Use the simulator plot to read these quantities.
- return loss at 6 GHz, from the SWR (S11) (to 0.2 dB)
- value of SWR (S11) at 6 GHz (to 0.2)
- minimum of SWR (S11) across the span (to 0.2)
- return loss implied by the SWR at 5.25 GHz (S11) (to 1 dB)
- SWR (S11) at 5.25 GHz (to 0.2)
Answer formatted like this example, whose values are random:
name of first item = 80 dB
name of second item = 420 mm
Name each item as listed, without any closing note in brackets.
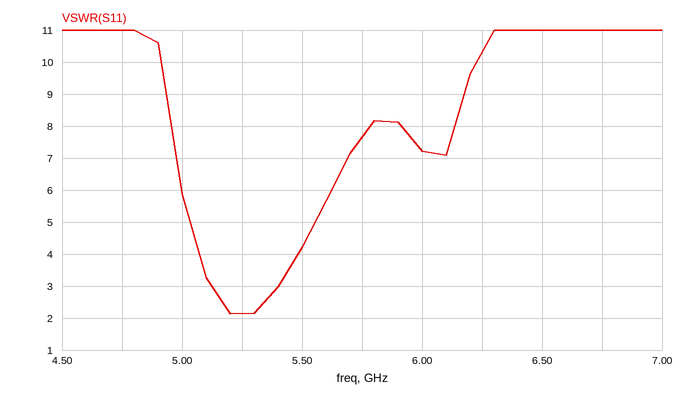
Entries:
return loss at 6 GHz, from the SWR (S11) = 2.4 dB
value of SWR (S11) at 6 GHz = 7.2
minimum of SWR (S11) across the span = 2.2
return loss implied by the SWR at 5.25 GHz (S11) = 9 dB
SWR (S11) at 5.25 GHz = 2.2
